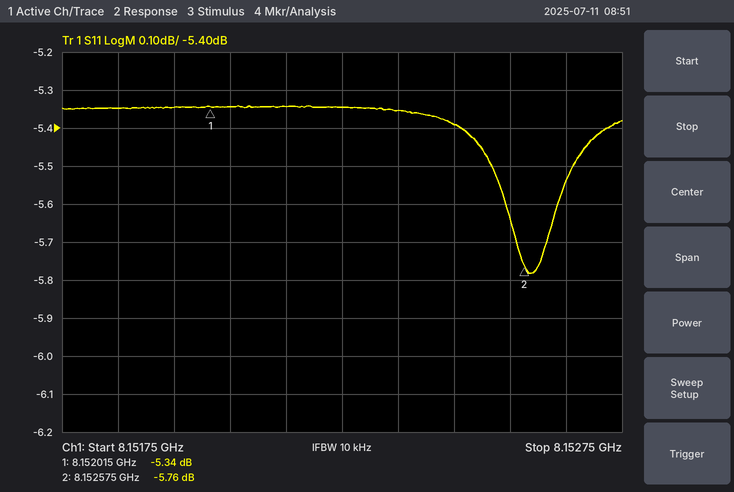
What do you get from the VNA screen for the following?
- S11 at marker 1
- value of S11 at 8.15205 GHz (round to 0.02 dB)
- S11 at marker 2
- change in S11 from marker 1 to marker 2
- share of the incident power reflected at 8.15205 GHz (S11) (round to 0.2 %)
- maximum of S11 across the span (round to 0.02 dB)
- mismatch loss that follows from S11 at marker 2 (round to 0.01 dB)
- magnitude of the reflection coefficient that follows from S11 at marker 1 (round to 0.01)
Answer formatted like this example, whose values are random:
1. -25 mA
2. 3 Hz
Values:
1. -5.34 dB
2. -5.34 dB
3. -5.76 dB
4. -0.42 dB
5. 29.2 %
6. -5.34 dB
7. 1.34 dB
8. 0.54
